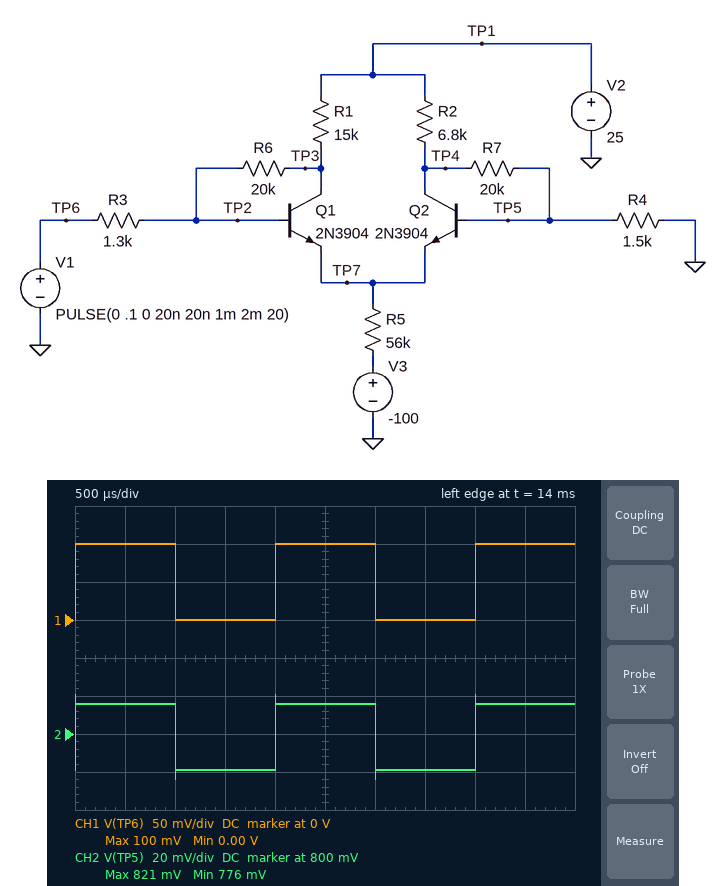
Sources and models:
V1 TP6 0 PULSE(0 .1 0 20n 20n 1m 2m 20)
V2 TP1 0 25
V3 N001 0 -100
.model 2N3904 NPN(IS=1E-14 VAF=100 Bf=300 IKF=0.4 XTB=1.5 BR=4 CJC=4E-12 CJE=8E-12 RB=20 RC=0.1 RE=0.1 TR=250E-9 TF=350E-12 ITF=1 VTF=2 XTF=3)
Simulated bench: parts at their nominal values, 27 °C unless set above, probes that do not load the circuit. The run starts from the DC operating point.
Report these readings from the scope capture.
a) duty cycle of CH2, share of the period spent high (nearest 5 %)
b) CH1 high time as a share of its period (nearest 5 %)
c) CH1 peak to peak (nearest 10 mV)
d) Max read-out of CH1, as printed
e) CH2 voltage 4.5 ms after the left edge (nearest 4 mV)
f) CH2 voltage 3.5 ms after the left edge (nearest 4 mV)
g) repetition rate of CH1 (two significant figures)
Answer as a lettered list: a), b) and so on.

a) 50 %
b) 50 %
c) 100 mV
d) 100 mV
e) 816 mV
f) 780 mV
g) 500 Hz
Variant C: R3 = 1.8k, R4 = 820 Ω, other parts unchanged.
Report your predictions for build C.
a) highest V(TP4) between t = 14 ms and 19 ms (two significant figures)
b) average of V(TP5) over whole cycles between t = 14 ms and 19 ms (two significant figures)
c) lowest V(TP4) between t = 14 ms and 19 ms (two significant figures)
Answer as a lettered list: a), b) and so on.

a) 15 V
b) 570 mV
c) 14 V
